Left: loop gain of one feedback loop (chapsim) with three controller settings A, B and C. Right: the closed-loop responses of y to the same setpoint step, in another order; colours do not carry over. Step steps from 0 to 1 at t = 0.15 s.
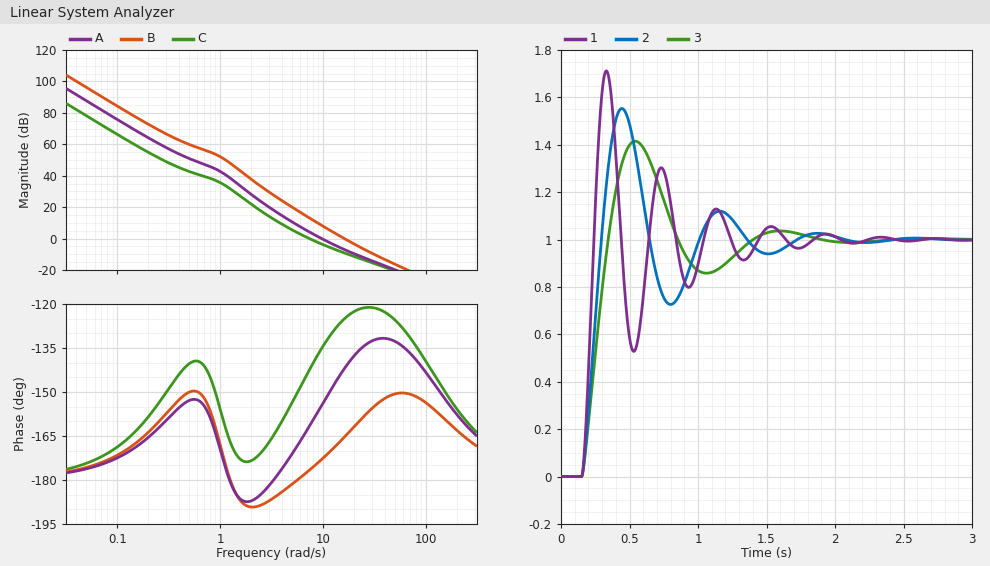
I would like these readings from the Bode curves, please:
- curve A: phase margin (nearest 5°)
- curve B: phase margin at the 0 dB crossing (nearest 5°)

25°
15°
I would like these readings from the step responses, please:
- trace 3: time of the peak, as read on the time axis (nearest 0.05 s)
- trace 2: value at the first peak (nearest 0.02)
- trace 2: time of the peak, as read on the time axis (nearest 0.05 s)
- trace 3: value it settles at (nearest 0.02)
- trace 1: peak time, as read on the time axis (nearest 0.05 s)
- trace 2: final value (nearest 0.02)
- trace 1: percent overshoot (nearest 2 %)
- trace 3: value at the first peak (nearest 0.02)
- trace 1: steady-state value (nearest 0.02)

0.55 s
1.56
0.45 s
1.00
0.35 s
1.00
72 %
1.42
1.00
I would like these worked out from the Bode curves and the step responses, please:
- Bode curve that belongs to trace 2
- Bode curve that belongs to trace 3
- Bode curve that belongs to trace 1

A
C
B
